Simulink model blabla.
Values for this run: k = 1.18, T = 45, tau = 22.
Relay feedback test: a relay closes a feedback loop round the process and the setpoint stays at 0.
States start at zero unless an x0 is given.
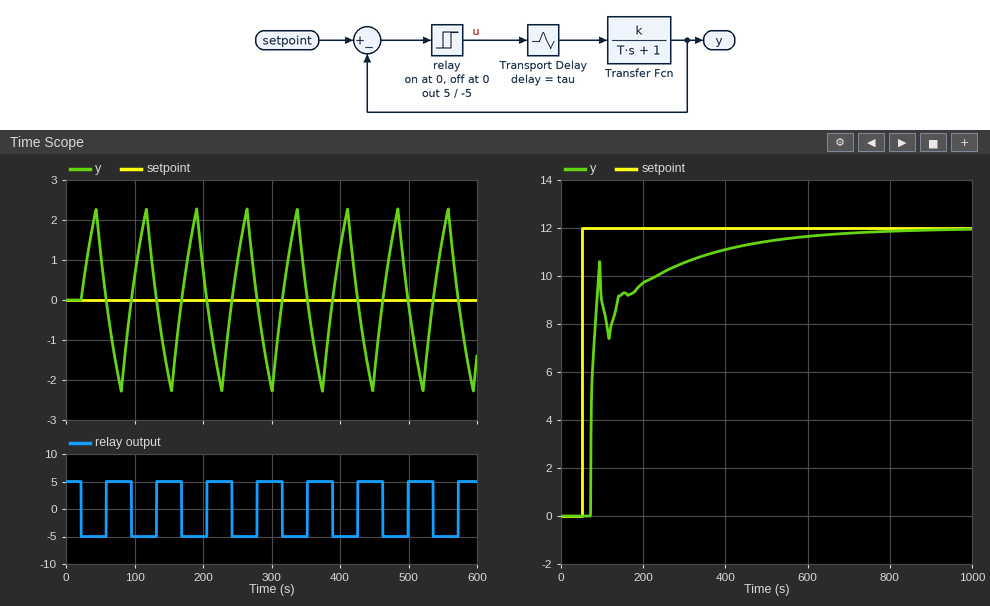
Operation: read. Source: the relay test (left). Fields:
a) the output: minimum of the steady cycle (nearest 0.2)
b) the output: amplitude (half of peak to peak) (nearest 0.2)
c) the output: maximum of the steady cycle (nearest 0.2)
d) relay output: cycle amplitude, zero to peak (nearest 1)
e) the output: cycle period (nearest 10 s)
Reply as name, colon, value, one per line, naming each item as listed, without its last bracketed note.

the output: minimum of the steady cycle: -2.2
the output: amplitude (half of peak to peak): 2.2
the output: maximum of the steady cycle: 2.2
relay output: cycle amplitude, zero to peak: 5
the output: cycle period: 70 s
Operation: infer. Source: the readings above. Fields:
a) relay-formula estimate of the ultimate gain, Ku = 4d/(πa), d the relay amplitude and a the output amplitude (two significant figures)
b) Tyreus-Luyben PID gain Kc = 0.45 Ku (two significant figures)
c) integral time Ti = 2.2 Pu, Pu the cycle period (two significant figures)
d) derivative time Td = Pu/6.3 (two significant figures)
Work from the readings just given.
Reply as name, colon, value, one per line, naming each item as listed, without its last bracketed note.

relay-formula estimate of the ultimate gain, Ku = 4d/(πa), d the relay amplitude and a the output amplitude: 2.9
Tyreus-Luyben PID gain Kc = 0.45 Ku: 1.3
integral time Ti = 2.2 Pu, Pu the cycle period: 150 s
derivative time Td = Pu/6.3: 11 s
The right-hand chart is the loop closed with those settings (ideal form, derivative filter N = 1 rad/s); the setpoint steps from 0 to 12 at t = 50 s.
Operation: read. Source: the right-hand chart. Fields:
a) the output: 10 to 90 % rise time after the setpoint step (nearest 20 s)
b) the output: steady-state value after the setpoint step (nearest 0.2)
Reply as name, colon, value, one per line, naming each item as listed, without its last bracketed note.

the output: 10 to 90 % rise time after the setpoint step: 260 s
the output: steady-state value after the setpoint step: 12.0
